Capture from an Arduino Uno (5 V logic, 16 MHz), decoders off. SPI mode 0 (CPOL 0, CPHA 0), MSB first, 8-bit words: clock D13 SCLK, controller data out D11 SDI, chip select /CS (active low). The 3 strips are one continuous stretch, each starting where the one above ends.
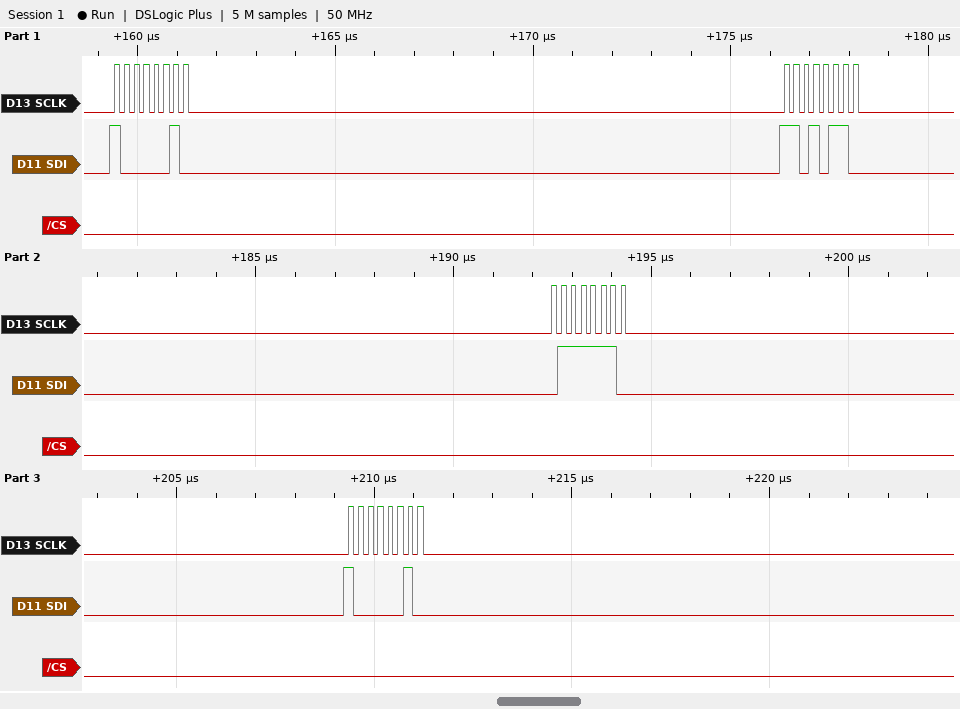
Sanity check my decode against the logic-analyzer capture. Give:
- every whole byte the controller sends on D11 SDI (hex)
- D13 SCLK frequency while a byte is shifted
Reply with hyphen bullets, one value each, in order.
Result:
- 82 D6 7E 82
- 4 MHz
